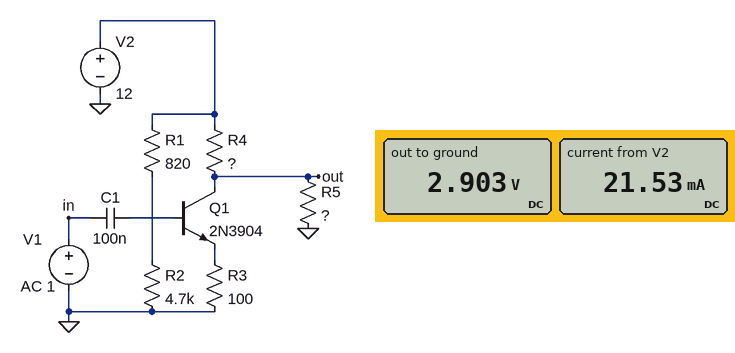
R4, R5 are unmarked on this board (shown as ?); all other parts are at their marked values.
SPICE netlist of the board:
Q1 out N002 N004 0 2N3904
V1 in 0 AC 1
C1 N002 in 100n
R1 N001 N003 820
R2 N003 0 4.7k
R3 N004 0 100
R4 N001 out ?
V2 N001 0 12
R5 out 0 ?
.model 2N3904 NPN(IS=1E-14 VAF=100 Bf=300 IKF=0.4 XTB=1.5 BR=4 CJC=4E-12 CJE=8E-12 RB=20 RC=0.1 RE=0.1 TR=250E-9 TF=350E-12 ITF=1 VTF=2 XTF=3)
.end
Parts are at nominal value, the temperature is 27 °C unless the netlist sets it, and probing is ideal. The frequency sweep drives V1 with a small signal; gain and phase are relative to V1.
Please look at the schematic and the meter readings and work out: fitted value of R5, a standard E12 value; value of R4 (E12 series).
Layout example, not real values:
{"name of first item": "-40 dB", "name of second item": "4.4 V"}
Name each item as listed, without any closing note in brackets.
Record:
{"fitted value of R5, a standard E12 value": "150 Ω", "value of R4": "470 Ω"}
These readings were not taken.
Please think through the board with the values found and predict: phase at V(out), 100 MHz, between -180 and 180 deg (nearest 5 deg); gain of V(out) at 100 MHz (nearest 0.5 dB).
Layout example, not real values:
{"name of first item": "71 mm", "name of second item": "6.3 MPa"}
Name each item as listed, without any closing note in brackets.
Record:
{"phase at V(out), 100 MHz, between -180 and 180 deg": "75 deg", "gain of V(out) at 100 MHz": "-16.0 dB"}
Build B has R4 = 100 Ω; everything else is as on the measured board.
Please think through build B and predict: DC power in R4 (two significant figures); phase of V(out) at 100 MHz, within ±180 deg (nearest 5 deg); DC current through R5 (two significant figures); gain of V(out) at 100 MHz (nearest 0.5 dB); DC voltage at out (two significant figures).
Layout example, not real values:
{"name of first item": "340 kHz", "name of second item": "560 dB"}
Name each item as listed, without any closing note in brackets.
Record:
{"DC power in R4": "230 mW", "phase of V(out) at 100 MHz, within ±180 deg": "80 deg", "DC current through R5": "48 mA", "gain of V(out) at 100 MHz": "-23.5 dB", "DC voltage at out": "7.2 V"}
